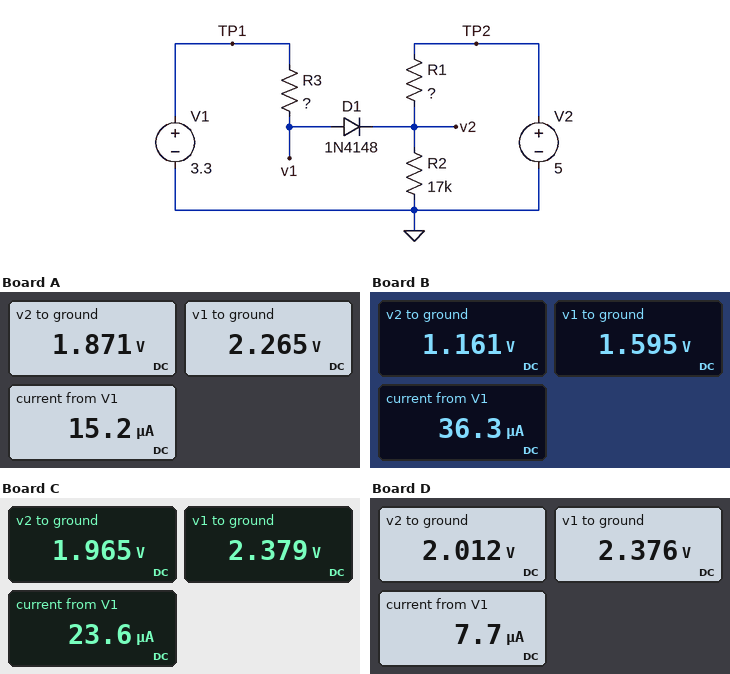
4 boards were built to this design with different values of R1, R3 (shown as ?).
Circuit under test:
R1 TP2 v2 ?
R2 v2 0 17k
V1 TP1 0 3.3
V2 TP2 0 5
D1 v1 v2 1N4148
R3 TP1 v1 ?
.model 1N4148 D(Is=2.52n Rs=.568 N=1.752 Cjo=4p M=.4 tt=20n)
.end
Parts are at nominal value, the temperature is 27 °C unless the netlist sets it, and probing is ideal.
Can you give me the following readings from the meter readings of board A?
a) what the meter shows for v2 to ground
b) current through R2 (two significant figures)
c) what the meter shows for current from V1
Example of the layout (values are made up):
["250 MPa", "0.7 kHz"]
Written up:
["1.871 V", "110 µA", "15.2 µA"]
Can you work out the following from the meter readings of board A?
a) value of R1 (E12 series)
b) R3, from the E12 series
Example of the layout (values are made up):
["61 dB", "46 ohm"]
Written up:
["33 kΩ", "68 kΩ"]
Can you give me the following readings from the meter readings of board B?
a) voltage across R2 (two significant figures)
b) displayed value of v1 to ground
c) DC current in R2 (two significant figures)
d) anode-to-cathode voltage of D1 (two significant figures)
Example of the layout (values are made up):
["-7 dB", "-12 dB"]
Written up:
["1.2 V", "1.595 V", "68 µA", "430 mV"]
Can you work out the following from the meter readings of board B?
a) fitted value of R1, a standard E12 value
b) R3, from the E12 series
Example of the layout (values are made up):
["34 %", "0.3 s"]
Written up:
["120 kΩ", "47 kΩ"]
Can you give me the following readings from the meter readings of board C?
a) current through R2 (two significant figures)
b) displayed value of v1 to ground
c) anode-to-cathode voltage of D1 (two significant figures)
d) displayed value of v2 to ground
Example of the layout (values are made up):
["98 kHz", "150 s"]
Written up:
["120 µA", "2.379 V", "410 mV", "1.965 V"]
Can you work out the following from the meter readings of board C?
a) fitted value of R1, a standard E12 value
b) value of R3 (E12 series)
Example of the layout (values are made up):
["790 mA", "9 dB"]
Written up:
["33 kΩ", "39 kΩ"]
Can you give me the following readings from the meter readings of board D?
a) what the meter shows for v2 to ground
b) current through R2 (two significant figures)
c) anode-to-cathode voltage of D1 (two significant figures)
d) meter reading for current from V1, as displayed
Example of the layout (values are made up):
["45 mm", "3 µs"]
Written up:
["2.012 V", "120 µA", "360 mV", "7.7 µA"]
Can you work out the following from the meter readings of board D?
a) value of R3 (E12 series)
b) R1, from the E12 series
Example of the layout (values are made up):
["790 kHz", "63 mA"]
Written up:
["120 kΩ", "27 kΩ"]
